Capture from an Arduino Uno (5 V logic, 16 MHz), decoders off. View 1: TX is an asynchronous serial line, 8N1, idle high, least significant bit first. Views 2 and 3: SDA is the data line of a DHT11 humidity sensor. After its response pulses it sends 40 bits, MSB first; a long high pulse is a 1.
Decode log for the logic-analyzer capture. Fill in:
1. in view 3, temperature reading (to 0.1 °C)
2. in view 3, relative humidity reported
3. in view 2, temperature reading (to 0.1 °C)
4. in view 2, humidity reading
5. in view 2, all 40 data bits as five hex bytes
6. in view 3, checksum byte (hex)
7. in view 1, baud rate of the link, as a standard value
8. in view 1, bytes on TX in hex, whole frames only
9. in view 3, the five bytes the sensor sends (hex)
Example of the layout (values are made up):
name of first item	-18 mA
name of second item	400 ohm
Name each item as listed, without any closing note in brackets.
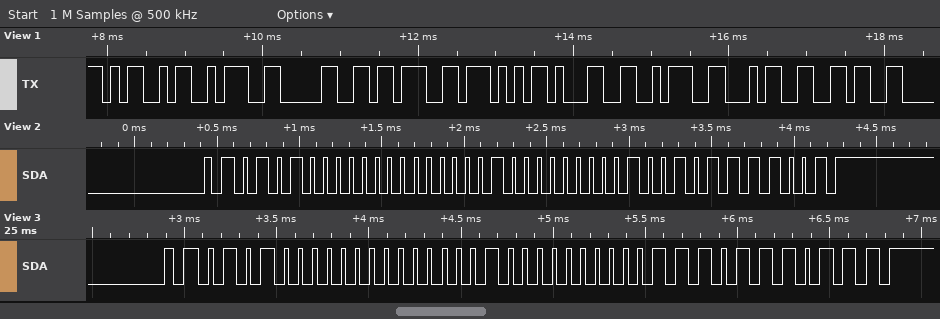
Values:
in view 3, temperature reading	32.7 °C
in view 3, relative humidity reported	80 %
in view 2, temperature reading	32.9 °C
in view 2, humidity reading	80 %
in view 2, all 40 data bits as five hex bytes	50 00 20 09 79
in view 3, checksum byte	0x77
in view 1, baud rate of the link, as a standard value	9600 baud
in view 1, bytes on TX in hex, whole frames only	4D 3A 30 3B 57 31 3A 34 36
in view 3, the five bytes the sensor sends	50 00 20 07 77
